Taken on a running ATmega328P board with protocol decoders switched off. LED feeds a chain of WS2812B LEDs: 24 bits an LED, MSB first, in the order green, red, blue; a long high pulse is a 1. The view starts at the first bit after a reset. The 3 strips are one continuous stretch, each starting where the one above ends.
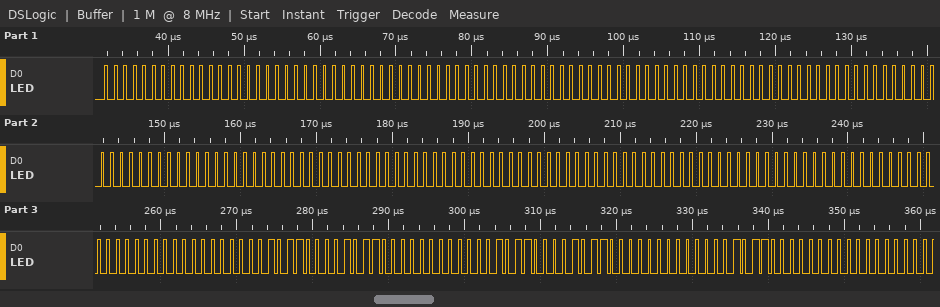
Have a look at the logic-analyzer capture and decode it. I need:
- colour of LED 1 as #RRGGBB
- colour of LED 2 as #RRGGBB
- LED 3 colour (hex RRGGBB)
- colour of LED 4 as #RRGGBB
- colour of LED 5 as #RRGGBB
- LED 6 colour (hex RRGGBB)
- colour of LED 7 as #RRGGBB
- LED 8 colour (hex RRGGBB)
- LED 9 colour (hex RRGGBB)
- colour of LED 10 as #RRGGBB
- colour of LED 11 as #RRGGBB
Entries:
#000000
#000000
#000000
#000000
#000000
#000000
#000000
#000000
#2C2C00
#2C2C00
#001600
